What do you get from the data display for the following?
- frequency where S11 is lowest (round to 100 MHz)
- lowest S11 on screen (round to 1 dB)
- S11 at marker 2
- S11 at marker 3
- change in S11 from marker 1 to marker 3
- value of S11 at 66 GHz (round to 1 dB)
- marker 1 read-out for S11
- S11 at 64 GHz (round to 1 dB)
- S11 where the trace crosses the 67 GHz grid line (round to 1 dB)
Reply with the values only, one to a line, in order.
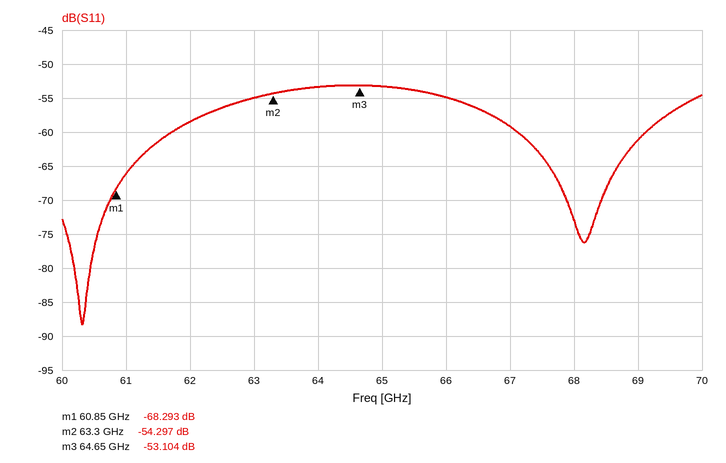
60.3 GHz
-88 dB
-54.297 dB
-53.104 dB
15.189 dB
-55 dB
-68.293 dB
-53 dB
-59 dB
